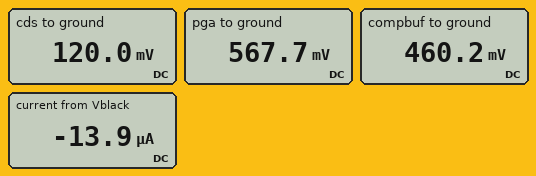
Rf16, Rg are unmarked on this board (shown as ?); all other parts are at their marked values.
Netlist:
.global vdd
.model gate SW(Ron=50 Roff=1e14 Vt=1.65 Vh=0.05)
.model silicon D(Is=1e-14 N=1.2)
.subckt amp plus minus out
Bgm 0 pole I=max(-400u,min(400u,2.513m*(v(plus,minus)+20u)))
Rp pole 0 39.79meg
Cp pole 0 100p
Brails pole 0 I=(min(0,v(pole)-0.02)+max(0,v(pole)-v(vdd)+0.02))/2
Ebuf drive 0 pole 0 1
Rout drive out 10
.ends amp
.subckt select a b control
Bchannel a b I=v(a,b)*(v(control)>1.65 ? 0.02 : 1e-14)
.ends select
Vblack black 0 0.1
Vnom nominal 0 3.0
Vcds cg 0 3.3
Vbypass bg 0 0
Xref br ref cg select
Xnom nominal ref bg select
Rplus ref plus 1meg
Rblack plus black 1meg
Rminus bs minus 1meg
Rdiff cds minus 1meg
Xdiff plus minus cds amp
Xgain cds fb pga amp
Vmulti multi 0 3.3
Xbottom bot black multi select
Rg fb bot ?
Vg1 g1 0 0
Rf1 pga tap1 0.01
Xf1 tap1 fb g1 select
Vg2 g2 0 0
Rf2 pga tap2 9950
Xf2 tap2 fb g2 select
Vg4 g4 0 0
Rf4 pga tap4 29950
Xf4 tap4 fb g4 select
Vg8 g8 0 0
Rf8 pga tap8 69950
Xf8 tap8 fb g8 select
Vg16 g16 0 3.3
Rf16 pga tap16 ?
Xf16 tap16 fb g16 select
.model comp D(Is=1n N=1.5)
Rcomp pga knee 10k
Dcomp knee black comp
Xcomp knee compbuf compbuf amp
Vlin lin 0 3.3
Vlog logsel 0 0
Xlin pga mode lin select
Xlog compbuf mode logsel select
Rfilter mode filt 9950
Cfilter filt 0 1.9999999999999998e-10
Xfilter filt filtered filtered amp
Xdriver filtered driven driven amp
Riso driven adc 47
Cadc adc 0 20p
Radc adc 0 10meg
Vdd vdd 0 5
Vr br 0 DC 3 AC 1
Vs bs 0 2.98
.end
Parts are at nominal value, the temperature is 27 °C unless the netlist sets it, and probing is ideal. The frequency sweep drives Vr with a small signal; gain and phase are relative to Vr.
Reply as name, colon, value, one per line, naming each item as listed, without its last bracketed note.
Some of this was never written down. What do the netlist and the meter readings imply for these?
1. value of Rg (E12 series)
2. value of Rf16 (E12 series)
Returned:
value of Rg: 12 kΩ
value of Rf16: 270 kΩ
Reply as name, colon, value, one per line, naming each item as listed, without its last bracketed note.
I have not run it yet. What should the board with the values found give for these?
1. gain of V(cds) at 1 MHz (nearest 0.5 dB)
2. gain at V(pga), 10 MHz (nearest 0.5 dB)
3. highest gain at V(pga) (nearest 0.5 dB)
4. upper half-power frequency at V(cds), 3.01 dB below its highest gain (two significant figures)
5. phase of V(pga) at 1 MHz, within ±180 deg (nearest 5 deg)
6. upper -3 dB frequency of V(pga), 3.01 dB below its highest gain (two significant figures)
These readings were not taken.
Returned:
gain of V(cds) at 1 MHz: -1.0 dB
gain at V(pga), 10 MHz: -22.0 dB
highest gain at V(pga): 27.5 dB
upper half-power frequency at V(cds), 3.01 dB below its highest gain: 2.0 MHz
phase of V(pga) at 1 MHz, within ±180 deg: -105 deg
upper -3 dB frequency of V(pga), 3.01 dB below its highest gain: 170 kHz
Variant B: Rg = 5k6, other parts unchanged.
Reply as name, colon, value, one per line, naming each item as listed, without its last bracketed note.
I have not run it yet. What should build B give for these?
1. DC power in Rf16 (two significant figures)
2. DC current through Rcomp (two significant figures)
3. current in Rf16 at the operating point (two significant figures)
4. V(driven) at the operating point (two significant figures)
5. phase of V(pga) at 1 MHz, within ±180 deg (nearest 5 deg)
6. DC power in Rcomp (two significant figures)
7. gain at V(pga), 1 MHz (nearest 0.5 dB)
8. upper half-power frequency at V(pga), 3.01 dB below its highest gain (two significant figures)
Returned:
DC power in Rf16: 3.4 µW
DC current through Rcomp: 55 µA
current in Rf16 at the operating point: 3.5 µA
V(driven) at the operating point: 1.1 V
phase of V(pga) at 1 MHz, within ±180 deg: -110 deg
DC power in Rcomp: 30 µW
gain at V(pga), 1 MHz: 11.0 dB
upper half-power frequency at V(pga), 3.01 dB below its highest gain: 82 kHz
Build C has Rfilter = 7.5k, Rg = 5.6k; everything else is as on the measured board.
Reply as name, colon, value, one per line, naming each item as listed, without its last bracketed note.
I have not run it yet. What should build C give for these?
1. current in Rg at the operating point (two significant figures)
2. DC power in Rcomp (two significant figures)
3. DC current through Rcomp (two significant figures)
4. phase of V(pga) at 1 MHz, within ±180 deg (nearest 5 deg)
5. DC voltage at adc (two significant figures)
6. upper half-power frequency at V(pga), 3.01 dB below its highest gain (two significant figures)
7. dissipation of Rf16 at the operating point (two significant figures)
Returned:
current in Rg at the operating point: 3.5 µA
DC power in Rcomp: 30 µW
DC current through Rcomp: 55 µA
phase of V(pga) at 1 MHz, within ±180 deg: -110 deg
DC voltage at adc: 1.1 V
upper half-power frequency at V(pga), 3.01 dB below its highest gain: 82 kHz
dissipation of Rf16 at the operating point: 3.4 µW
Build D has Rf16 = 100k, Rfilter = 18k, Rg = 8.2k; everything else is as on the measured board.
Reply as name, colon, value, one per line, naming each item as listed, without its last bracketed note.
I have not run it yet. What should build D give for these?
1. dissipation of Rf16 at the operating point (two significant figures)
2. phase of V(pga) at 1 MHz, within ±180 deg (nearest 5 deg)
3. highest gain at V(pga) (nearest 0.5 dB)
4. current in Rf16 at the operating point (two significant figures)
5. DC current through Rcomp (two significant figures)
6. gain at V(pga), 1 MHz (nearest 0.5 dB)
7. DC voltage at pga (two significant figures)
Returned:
dissipation of Rf16 at the operating point: 590 nW
phase of V(pga) at 1 MHz, within ±180 deg: -100 deg
highest gain at V(pga): 22.5 dB
current in Rf16 at the operating point: 2.4 µA
DC current through Rcomp: 720 nA
gain at V(pga), 1 MHz: 10.5 dB
DC voltage at pga: 360 mV
